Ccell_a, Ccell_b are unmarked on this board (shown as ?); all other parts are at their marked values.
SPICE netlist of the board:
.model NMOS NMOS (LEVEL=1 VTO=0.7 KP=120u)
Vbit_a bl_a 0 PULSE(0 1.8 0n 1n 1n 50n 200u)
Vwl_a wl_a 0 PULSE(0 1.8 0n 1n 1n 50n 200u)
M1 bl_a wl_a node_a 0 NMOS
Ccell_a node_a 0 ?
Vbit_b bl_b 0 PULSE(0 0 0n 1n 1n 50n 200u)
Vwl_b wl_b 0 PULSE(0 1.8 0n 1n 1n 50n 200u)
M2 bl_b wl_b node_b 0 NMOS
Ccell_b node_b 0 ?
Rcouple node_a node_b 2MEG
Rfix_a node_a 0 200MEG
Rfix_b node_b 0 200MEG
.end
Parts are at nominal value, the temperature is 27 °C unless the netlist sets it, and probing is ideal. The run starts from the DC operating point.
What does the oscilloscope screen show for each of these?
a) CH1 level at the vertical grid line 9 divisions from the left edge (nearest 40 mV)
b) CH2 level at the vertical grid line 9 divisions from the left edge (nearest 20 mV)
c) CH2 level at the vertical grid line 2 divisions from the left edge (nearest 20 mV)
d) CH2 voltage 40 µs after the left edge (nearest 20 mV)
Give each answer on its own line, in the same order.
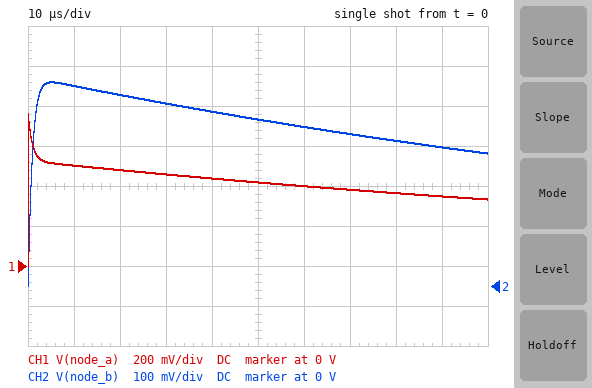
360 mV
340 mV
480 mV
440 mV
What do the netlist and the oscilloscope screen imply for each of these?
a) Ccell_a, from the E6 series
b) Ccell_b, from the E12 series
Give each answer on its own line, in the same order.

1.5 pF
680 fF
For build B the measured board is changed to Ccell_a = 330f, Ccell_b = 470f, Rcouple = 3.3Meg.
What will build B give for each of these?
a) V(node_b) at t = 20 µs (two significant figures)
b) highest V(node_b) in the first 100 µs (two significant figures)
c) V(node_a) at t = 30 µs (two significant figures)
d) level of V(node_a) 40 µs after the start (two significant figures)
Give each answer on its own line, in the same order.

320 mV
390 mV
280 mV
250 mV
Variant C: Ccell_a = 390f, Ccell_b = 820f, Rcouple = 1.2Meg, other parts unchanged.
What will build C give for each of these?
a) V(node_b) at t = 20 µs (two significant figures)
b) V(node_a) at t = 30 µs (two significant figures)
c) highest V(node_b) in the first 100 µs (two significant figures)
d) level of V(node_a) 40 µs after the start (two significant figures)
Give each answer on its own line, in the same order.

260 mV
240 mV
310 mV
220 mV
